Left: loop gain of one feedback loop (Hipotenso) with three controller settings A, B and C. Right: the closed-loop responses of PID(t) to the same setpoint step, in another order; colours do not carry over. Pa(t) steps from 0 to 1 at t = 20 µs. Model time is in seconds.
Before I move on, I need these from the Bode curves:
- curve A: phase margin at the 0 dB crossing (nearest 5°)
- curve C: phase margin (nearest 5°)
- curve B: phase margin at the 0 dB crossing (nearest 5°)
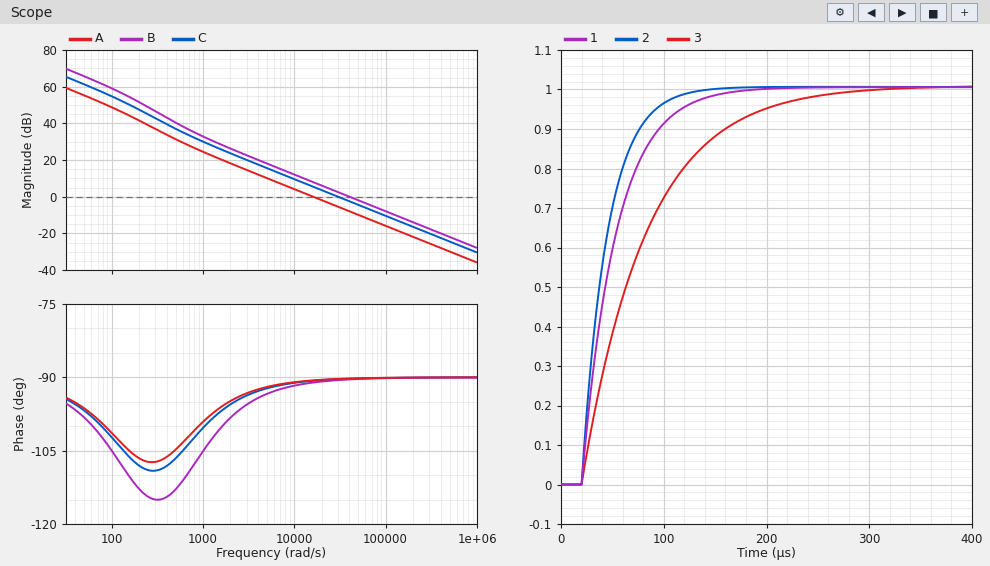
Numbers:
90°
90°
90°
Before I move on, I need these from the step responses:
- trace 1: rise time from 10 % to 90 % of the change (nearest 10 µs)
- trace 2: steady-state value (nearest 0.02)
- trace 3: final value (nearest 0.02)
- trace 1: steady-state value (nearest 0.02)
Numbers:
70 µs
1.00
1.00
1.00
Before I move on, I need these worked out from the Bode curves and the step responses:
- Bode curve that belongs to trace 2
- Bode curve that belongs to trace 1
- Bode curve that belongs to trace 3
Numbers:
B
C
A
